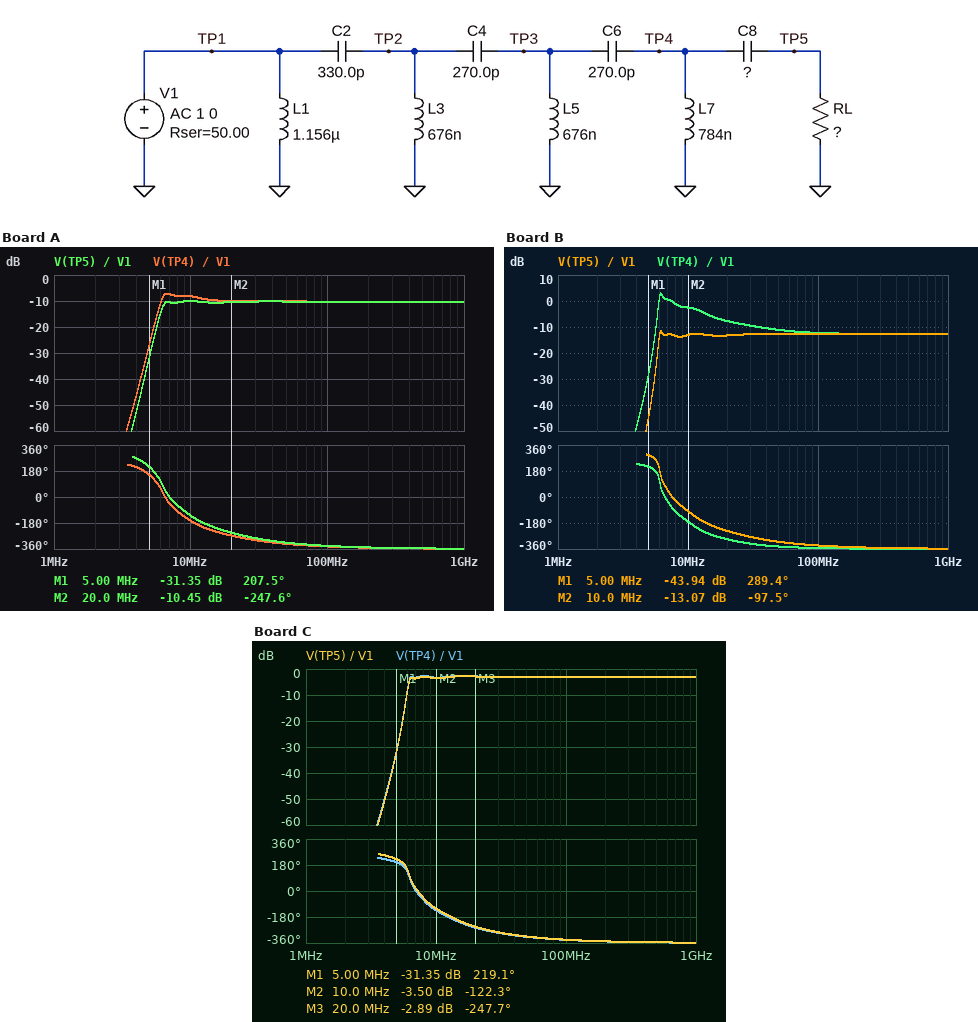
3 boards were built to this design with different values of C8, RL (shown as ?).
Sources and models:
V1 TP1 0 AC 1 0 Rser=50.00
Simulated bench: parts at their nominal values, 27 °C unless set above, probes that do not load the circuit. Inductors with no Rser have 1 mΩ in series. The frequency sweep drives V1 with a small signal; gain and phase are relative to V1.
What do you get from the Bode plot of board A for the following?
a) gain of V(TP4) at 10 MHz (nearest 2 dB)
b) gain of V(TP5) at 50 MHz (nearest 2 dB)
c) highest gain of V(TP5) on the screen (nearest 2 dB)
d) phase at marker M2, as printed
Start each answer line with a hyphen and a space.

- -8 dB
- -10 dB
- -10 dB
- -247.6 deg
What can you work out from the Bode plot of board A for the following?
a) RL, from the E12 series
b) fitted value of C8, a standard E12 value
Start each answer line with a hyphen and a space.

- 22 Ω
- 1 nF
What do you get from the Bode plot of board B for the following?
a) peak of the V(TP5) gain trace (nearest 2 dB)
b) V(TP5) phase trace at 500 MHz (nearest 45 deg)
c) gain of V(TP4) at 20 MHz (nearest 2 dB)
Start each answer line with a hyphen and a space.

- -12 dB
- -360 deg
- -8 dB
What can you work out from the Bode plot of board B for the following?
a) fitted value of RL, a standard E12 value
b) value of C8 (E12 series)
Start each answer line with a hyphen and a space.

- 15 Ω
- 330 pF
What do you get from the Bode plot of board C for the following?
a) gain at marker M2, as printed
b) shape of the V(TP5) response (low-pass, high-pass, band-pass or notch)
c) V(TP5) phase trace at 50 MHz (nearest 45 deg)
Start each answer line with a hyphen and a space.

- -3.50 dB
- high-pass
- -315 deg
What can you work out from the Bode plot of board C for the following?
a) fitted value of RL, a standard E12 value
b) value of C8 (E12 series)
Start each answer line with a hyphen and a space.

- 120 Ω
- 680 pF
